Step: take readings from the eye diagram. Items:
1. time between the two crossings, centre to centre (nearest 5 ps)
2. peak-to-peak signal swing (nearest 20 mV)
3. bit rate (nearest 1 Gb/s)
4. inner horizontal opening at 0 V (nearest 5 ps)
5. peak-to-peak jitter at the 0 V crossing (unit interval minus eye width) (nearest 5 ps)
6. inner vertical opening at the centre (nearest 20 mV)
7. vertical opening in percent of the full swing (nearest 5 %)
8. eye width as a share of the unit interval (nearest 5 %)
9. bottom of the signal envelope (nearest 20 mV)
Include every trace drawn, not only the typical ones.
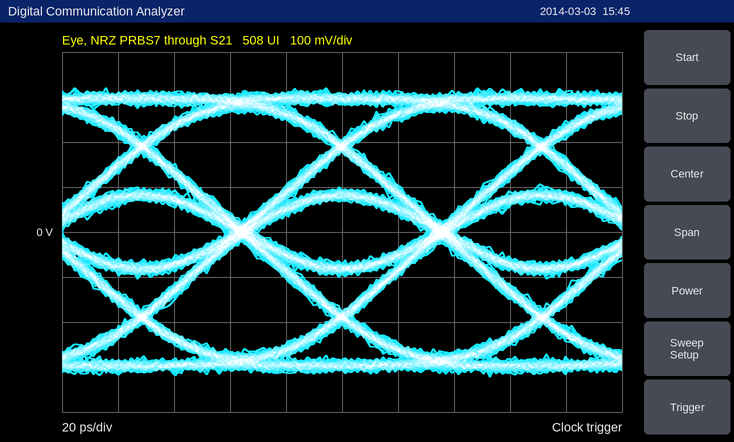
70 ps
640 mV
14 Gb/s
60 ps
10 ps
140 mV
20 %
85 %
-320 mV
